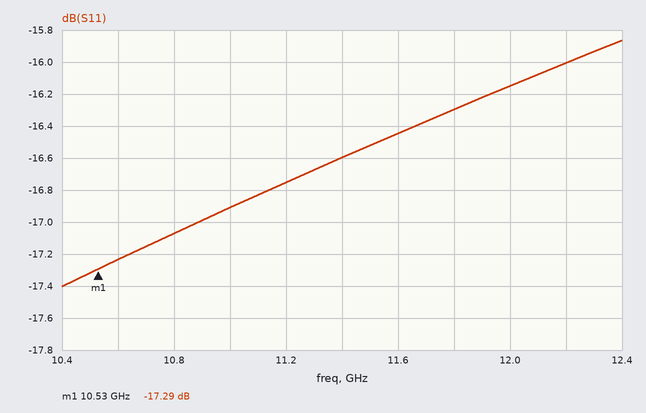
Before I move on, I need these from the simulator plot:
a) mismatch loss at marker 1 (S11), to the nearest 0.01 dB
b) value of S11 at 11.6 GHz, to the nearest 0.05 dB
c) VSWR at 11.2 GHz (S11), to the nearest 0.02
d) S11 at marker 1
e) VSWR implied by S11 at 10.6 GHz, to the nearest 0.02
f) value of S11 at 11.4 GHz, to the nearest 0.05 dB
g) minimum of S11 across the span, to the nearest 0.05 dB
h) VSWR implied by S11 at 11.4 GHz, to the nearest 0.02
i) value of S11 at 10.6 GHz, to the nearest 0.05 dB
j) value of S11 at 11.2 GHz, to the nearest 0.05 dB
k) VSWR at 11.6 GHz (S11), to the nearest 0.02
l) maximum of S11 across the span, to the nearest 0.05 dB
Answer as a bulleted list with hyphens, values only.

- 0.08 dB
- -16.45 dB
- 1.34
- -17.29 dB
- 1.32
- -16.60 dB
- -17.40 dB
- 1.34
- -17.25 dB
- -16.75 dB
- 1.36
- -15.85 dB
